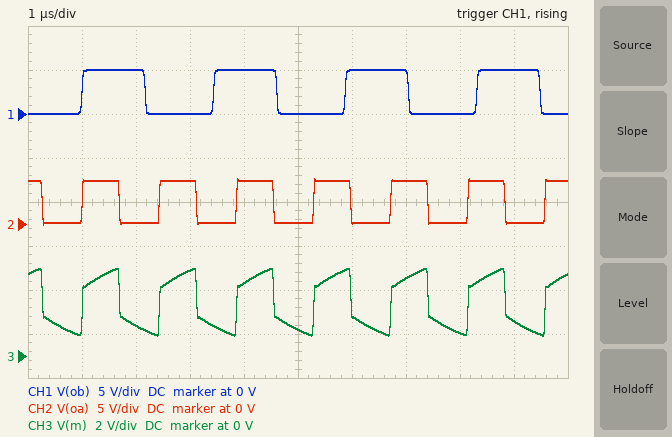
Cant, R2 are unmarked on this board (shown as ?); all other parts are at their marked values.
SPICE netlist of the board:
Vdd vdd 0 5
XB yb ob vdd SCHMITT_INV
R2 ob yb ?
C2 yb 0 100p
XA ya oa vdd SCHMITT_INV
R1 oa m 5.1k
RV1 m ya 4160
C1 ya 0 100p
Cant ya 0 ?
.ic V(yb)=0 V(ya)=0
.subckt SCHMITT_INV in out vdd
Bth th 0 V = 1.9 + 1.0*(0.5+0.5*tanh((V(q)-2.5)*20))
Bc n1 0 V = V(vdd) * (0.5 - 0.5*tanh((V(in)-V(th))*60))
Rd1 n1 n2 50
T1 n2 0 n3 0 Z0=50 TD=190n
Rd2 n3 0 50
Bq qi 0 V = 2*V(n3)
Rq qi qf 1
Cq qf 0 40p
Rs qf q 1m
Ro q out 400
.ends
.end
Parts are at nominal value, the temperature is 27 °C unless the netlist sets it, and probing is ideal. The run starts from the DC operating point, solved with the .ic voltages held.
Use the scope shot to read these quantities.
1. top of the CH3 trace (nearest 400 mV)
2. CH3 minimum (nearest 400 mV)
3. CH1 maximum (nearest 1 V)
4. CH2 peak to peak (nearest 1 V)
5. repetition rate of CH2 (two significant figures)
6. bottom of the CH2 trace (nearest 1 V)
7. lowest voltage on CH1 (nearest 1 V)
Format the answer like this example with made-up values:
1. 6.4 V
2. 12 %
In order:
1. 4.0 V
2. 800 mV
3. 5 V
4. 5 V
5. 700 kHz
6. 0 V
7. 0 V
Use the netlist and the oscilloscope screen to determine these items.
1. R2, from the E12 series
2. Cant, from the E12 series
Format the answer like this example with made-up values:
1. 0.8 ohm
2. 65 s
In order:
1. 22 kΩ
2. 5.6 pF
